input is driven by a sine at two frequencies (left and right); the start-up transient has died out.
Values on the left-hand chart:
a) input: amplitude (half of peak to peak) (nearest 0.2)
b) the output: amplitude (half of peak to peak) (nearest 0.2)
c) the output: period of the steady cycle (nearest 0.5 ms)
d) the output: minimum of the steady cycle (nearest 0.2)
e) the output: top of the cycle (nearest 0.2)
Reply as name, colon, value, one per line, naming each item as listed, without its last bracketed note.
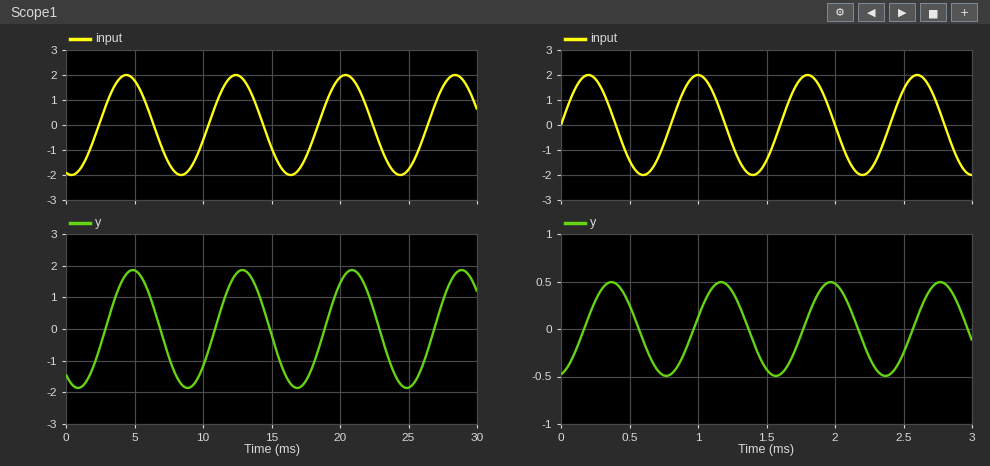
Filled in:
input: amplitude (half of peak to peak): 2.0
the output: amplitude (half of peak to peak): 1.8
the output: period of the steady cycle: 8.0 ms
the output: minimum of the steady cycle: -1.8
the output: top of the cycle: 1.8
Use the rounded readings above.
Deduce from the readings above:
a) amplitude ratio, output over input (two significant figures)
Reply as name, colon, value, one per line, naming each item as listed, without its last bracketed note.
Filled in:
amplitude ratio, output over input: 0.90
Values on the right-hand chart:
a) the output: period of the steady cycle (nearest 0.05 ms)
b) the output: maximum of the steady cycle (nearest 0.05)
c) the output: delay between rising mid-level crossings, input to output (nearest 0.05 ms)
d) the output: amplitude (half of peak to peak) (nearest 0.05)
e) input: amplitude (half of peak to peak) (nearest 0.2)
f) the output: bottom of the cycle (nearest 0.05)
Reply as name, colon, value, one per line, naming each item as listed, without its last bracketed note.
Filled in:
the output: period of the steady cycle: 0.80 ms
the output: maximum of the steady cycle: 0.50
the output: delay between rising mid-level crossings, input to output: 0.15 ms
the output: amplitude (half of peak to peak): 0.50
input: amplitude (half of peak to peak): 2.0
the output: bottom of the cycle: -0.50
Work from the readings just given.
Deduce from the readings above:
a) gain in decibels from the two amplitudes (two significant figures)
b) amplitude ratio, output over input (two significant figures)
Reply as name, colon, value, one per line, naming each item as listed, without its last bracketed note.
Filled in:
gain in decibels from the two amplitudes: -12 dB
amplitude ratio, output over input: 0.25
